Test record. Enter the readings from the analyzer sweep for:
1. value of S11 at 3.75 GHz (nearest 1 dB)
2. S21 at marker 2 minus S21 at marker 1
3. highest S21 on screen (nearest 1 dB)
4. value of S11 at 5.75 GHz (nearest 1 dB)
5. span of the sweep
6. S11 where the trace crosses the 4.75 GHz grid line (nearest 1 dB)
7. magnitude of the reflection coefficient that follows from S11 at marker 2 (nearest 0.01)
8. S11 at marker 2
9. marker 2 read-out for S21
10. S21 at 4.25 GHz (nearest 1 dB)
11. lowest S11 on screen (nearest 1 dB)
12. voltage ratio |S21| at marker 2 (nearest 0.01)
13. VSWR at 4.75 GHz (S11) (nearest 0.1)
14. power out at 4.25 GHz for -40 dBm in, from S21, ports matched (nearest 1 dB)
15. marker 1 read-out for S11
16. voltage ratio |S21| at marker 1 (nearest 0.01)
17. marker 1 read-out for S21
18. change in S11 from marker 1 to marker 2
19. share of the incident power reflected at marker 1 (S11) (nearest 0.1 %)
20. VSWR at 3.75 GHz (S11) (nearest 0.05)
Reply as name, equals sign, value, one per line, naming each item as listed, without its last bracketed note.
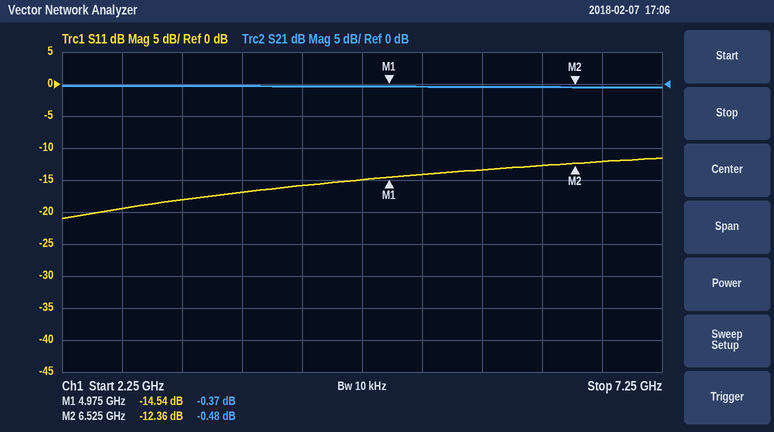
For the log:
value of S11 at 3.75 GHz = -17 dB
S21 at marker 2 minus S21 at marker 1 = -0.11 dB
highest S21 on screen = 0 dB
value of S11 at 5.75 GHz = -13 dB
span of the sweep = 5 GHz
S11 where the trace crosses the 4.75 GHz grid line = -15 dB
magnitude of the reflection coefficient that follows from S11 at marker 2 = 0.24
S11 at marker 2 = -12.36 dB
marker 2 read-out for S21 = -0.48 dB
S21 at 4.25 GHz = 0 dB
lowest S11 on screen = -21 dB
voltage ratio |S21| at marker 2 = 0.95
VSWR at 4.75 GHz (S11) = 1.4
power out at 4.25 GHz for -40 dBm in, from S21, ports matched = -40 dBm
marker 1 read-out for S11 = -14.54 dB
voltage ratio |S21| at marker 1 = 0.96
marker 1 read-out for S21 = -0.37 dB
change in S11 from marker 1 to marker 2 = 2.18 dB
share of the incident power reflected at marker 1 (S11) = 3.5 %
VSWR at 3.75 GHz (S11) = 1.35
